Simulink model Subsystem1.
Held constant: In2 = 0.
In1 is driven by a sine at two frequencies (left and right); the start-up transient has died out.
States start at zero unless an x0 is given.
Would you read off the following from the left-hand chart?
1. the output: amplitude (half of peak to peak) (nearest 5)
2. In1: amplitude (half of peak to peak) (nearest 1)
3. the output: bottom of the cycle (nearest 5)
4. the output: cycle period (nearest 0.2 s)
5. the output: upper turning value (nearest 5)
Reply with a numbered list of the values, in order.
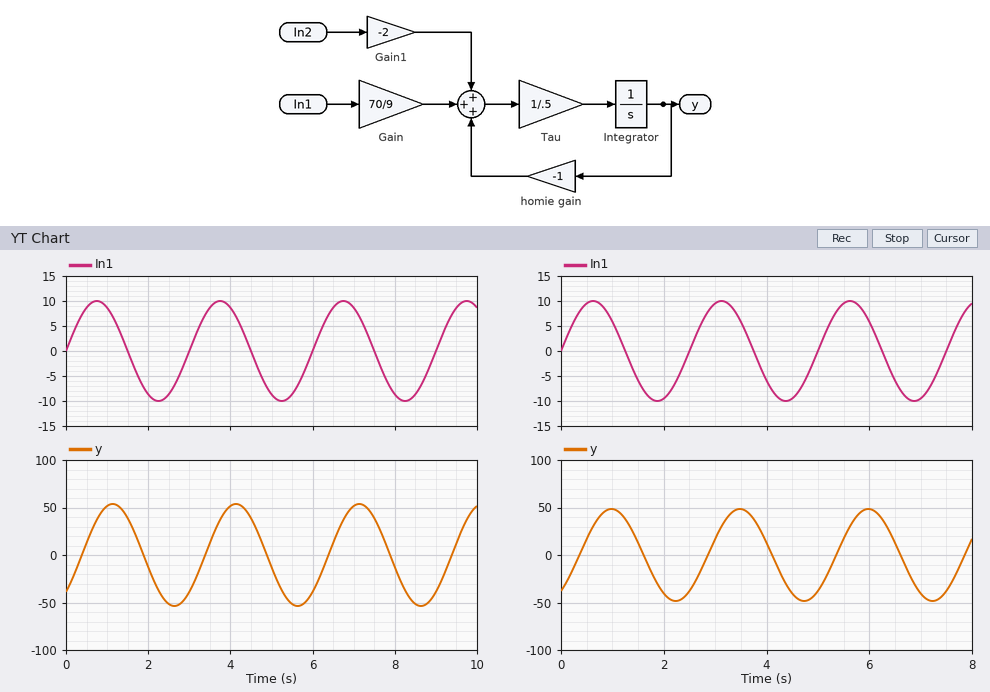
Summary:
1. 55
2. 10
3. -55
4. 3.0 s
5. 55
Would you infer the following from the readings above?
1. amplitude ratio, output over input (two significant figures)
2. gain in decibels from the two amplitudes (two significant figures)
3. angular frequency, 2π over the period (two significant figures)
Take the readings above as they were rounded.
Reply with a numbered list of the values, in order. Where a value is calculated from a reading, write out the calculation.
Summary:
1. 55 / 10 = 5.5
2. 20 log10(55 / 10) = 15 dB
3. 2π / 3 = 2.1 rad/s
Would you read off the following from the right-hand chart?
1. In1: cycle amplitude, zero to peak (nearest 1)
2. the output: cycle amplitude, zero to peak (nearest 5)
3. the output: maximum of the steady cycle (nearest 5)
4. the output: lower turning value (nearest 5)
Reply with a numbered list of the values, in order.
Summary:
1. 10
2. 50
3. 50
4. -50
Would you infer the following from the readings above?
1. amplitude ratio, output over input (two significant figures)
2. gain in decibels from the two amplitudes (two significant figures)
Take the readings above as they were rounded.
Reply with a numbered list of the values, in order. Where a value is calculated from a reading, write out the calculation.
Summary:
1. 50 / 10 = 5.0
2. 20 log10(50 / 10) = 14 dB
